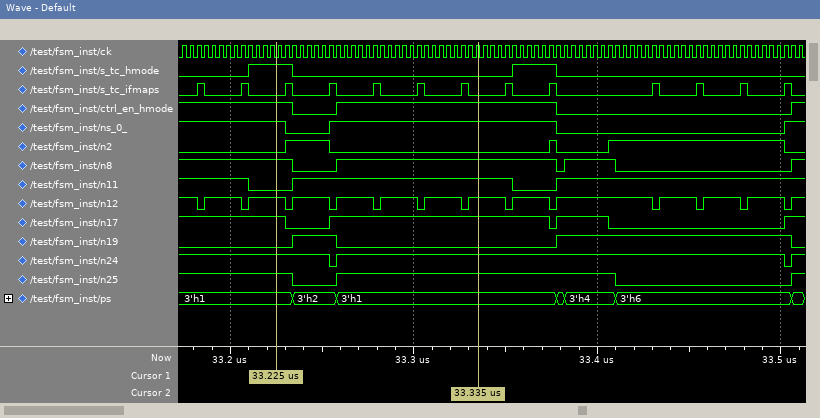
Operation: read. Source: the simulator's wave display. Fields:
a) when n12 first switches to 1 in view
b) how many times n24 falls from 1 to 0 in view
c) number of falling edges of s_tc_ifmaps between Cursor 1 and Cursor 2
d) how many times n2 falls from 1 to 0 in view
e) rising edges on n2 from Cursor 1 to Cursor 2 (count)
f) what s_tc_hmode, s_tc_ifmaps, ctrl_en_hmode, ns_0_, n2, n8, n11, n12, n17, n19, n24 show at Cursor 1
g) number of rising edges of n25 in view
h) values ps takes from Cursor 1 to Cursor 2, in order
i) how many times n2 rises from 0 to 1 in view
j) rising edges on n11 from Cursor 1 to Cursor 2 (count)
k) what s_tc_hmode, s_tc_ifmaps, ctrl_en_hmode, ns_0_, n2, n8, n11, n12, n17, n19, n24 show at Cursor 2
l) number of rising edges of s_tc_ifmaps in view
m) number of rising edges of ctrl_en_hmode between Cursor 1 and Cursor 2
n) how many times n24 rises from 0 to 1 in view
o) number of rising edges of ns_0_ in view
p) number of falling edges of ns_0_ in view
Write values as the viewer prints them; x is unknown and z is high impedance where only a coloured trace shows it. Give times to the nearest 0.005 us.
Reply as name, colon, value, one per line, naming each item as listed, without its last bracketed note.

when n12 first switches to 1 in view: 33.185 us
how many times n24 falls from 1 to 0 in view: 2
number of falling edges of s_tc_ifmaps between Cursor 1 and Cursor 2: 5
how many times n2 falls from 1 to 0 in view: 3
rising edges on n2 from Cursor 1 to Cursor 2: 1
what s_tc_hmode, s_tc_ifmaps, ctrl_en_hmode, ns_0_, n2, n8, n11, n12, n17, n19, n24 show at Cursor 1: s_tc_hmode=1, s_tc_ifmaps=0, ctrl_en_hmode=1, ns_0_=1, n2=0, n8=1, n11=0, n12=1, n17=1, n19=0, n24=1
number of rising edges of n25 in view: 2
values ps takes from Cursor 1 to Cursor 2, in order: 3'h1, 3'h2, 3'h1
how many times n2 rises from 0 to 1 in view: 3
rising edges on n11 from Cursor 1 to Cursor 2: 1
what s_tc_hmode, s_tc_ifmaps, ctrl_en_hmode, ns_0_, n2, n8, n11, n12, n17, n19, n24 show at Cursor 2: s_tc_hmode=0, s_tc_ifmaps=0, ctrl_en_hmode=1, ns_0_=1, n2=0, n8=1, n11=1, n12=1, n17=1, n19=0, n24=1
number of rising edges of s_tc_ifmaps in view: 13
number of rising edges of ctrl_en_hmode between Cursor 1 and Cursor 2: 1
how many times n24 rises from 0 to 1 in view: 2
number of rising edges of ns_0_ in view: 2
number of falling edges of ns_0_ in view: 2
